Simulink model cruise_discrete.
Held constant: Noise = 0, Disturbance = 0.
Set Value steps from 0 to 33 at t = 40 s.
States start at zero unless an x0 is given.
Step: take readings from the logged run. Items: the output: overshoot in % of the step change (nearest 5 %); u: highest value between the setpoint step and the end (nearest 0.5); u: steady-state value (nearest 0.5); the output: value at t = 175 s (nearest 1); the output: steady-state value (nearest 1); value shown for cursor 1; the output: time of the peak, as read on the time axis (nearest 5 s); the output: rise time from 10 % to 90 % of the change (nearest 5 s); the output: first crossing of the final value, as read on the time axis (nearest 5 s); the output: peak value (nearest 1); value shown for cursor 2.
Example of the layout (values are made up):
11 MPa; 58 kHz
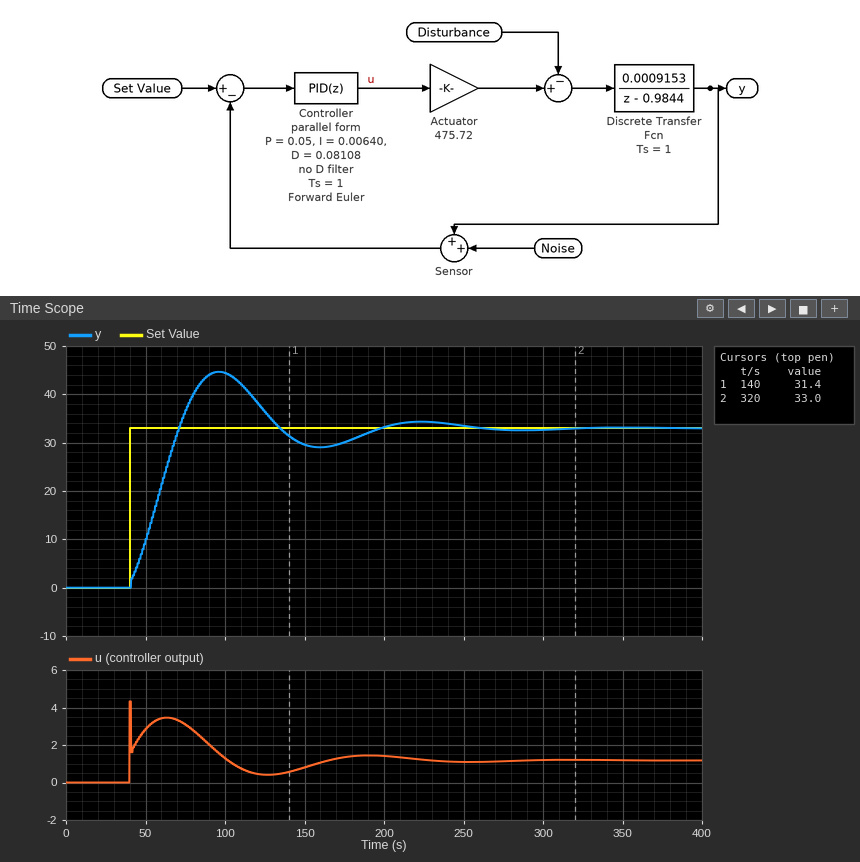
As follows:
35 %; 4.5; 1.0; 30; 33; 31.4; 95 s; 25 s; 70 s; 45; 33.0
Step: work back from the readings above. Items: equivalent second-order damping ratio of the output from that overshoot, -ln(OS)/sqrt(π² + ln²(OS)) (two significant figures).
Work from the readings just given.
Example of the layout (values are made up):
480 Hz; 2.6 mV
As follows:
0.32
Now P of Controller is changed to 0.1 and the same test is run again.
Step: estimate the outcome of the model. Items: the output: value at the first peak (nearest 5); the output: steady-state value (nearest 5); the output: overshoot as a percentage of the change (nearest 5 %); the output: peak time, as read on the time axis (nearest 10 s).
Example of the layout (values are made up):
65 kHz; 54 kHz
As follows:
40; 35; 20 %; 90 s
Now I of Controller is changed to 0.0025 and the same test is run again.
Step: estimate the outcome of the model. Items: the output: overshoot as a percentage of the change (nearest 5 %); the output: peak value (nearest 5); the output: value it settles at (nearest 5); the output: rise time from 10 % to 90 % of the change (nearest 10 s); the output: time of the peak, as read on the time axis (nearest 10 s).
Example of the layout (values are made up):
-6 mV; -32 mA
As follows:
15 %; 40; 35; 40 s; 130 s
